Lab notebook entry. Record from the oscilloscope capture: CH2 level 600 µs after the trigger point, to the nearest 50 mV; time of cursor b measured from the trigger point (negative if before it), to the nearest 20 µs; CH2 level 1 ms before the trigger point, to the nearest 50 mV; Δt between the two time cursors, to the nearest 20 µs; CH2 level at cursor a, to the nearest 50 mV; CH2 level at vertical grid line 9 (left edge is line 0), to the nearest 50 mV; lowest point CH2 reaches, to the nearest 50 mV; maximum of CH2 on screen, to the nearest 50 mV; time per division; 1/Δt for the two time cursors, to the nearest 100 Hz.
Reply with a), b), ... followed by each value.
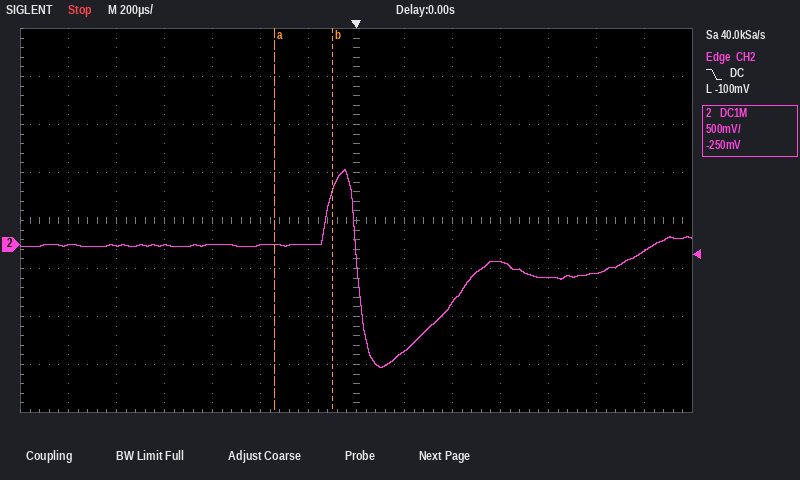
a) -200 mV
b) -100 µs
c) 0 mV
d) 240 µs
e) 0 mV
f) -600 mV
g) -1.30 V
h) 800 mV
i) 200 µs
j) 4.2 kHz
